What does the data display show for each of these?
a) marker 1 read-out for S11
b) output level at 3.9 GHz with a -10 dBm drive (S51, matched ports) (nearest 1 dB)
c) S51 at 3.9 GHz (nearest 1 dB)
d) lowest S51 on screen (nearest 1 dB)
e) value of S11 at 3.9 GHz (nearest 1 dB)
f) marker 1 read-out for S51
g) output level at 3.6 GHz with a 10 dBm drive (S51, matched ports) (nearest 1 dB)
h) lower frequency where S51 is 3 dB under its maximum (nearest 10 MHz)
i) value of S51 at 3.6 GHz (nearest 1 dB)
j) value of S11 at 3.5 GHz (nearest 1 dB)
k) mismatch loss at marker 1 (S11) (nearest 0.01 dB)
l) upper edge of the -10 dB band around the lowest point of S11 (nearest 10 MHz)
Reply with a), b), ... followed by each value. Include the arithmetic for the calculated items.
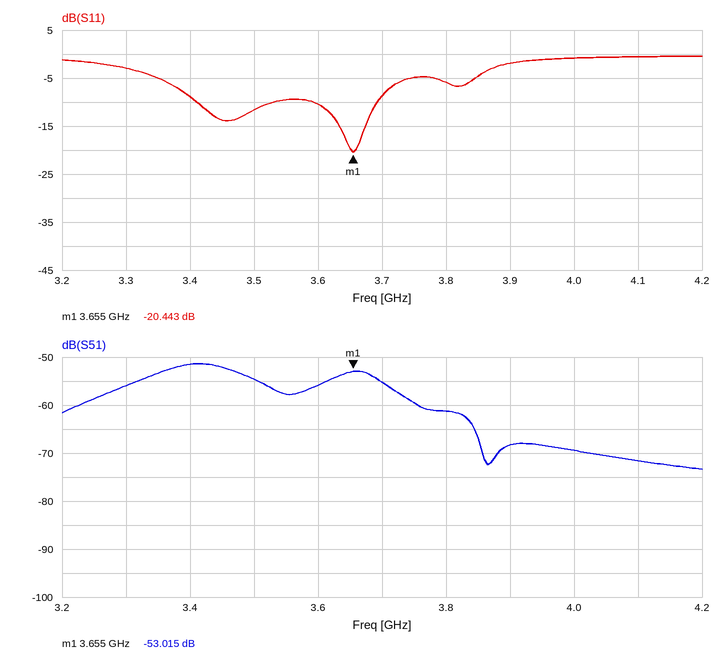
a) -20.443 dB
b) -10 dBm + (-68 dB) = -78 dBm
c) -68 dB
d) -73 dB
e) -2 dB
f) -53.015 dB
g) 10 dBm + (-56 dB) = -46 dBm
h) 3.33 GHz
i) -56 dB
j) -12 dB
k) −10 log10(1 − 10^(-20.443/10)) ≈ 0.04 dB
l) 3.69 GHz
